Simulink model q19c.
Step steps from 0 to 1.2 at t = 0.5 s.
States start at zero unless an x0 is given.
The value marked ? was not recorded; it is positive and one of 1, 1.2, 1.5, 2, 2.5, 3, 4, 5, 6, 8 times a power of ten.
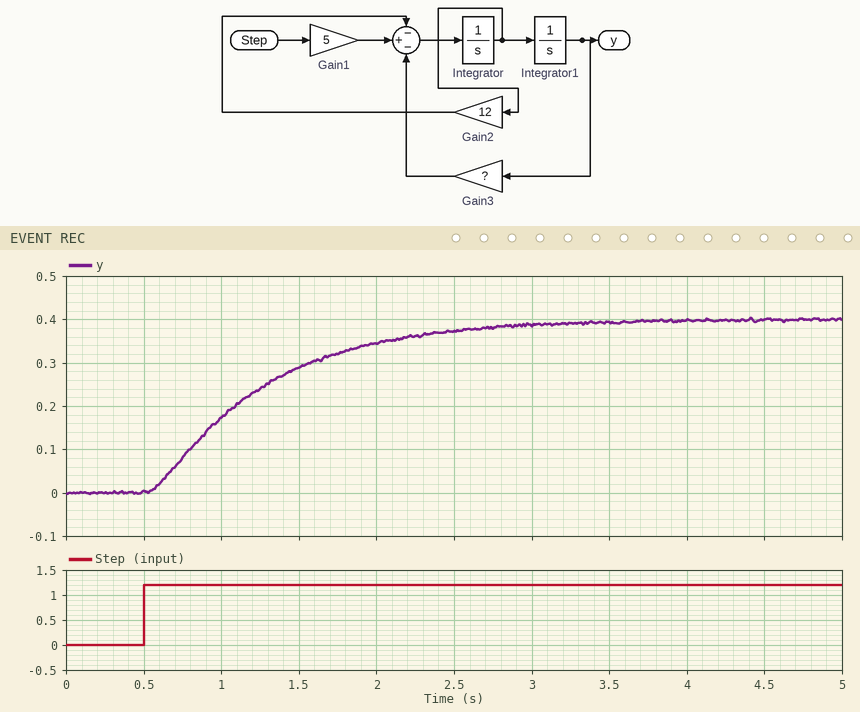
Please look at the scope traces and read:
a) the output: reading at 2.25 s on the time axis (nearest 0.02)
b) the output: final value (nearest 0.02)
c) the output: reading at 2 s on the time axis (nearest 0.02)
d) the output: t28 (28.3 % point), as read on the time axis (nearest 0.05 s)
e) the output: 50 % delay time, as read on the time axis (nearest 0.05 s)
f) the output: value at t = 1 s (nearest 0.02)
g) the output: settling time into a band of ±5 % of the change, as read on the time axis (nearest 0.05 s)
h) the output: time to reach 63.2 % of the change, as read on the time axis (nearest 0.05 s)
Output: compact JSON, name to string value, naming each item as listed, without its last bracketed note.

{"the output: reading at 2.25 s on the time axis": "0.36", "the output: final value": "0.40", "the output: reading at 2 s on the time axis": "0.34", "the output: t28 (28.3 % point), as read on the time axis": "0.85 s", "the output: 50 % delay time, as read on the time axis": "1.10 s", "the output: value at t = 1 s": "0.18", "the output: settling time into a band of ±5 % of the change, as read on the time axis": "2.70 s", "the output: time to reach 63.2 % of the change, as read on the time axis": "1.30 s"}
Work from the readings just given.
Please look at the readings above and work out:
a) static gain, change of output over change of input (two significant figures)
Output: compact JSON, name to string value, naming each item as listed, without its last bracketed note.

{"static gain, change of output over change of input": "0.33"}
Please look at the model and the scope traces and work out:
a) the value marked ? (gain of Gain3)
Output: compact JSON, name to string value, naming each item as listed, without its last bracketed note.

{"the value marked ?": "15"}
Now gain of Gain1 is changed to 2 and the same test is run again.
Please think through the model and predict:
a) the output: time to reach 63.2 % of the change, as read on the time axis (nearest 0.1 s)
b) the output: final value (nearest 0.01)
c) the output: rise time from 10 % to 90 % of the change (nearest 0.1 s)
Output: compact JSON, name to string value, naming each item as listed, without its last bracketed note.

{"the output: time to reach 63.2 % of the change, as read on the time axis": "1.3 s", "the output: final value": "0.16", "the output: rise time from 10 % to 90 % of the change": "1.6 s"}
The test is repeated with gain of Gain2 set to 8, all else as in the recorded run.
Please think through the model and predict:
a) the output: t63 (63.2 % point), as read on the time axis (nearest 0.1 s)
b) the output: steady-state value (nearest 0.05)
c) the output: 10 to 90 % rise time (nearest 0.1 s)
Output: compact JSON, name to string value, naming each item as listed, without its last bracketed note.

{"the output: t63 (63.2 % point), as read on the time axis": "1.1 s", "the output: steady-state value": "0.40", "the output: 10 to 90 % rise time": "0.9 s"}
